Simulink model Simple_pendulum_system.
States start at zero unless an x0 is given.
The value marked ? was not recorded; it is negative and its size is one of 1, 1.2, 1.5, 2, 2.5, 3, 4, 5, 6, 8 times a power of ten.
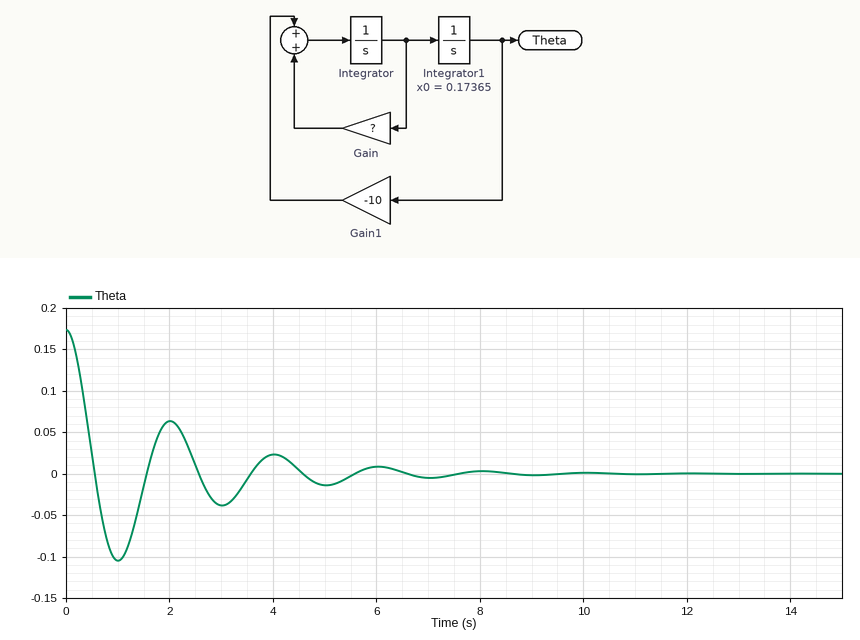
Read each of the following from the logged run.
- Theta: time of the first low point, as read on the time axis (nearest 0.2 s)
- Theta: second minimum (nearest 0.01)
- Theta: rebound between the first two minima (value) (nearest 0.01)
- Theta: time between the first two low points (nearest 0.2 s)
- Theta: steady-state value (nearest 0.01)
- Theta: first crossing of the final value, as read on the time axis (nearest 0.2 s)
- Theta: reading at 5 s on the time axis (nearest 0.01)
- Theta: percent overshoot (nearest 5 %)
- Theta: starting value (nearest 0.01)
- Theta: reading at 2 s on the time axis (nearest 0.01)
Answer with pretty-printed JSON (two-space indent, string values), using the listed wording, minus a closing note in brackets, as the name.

{
  "Theta: time of the first low point, as read on the time axis": "1.0 s",
  "Theta: second minimum": "-0.04",
  "Theta: rebound between the first two minima (value)": "0.06",
  "Theta: time between the first two low points": "2.0 s",
  "Theta: steady-state value": "0.00",
  "Theta: first crossing of the final value, as read on the time axis": "0.6 s",
  "Theta: reading at 5 s on the time axis": "-0.01",
  "Theta: percent overshoot": "60 %",
  "Theta: starting value": "0.17",
  "Theta: reading at 2 s on the time axis": "0.06"
}
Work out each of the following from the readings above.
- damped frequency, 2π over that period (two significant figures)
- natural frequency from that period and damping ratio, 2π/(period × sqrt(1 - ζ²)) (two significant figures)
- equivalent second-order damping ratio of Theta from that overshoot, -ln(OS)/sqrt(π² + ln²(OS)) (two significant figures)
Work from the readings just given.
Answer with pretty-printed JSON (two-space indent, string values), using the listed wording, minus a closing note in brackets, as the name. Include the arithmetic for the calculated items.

{
  "damped frequency, 2π over that period": "2π / 2 = 3.1 rad/s",
  "natural frequency from that period and damping ratio, 2π/(period × sqrt(1 - ζ²))": "2π / (2 × sqrt(1 - 0.16²)) = 3.2 rad/s",
  "equivalent second-order damping ratio of Theta from that overshoot, -ln(OS)/sqrt(π² + ln²(OS))": "ln(0.6) = -0.511; 0.511 / sqrt(9.870 + 0.261) = 0.16"
}
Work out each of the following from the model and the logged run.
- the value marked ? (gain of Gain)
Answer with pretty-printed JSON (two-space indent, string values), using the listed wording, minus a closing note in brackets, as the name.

{
  "the value marked ?": "-1"
}
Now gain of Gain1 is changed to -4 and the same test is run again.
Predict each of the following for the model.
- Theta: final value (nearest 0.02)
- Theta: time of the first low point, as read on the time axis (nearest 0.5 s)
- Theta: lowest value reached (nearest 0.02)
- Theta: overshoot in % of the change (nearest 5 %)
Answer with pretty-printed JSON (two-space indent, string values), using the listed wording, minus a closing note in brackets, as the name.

{
  "Theta: final value": "0.00",
  "Theta: time of the first low point, as read on the time axis": "1.5 s",
  "Theta: lowest value reached": "-0.08",
  "Theta: overshoot in % of the change": "45 %"
}
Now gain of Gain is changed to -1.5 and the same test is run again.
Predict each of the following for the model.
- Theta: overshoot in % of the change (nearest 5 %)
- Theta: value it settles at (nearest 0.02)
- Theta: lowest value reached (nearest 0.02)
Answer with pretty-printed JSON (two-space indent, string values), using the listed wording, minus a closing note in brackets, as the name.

{
  "Theta: overshoot in % of the change": "45 %",
  "Theta: value it settles at": "0.00",
  "Theta: lowest value reached": "-0.08"
}
